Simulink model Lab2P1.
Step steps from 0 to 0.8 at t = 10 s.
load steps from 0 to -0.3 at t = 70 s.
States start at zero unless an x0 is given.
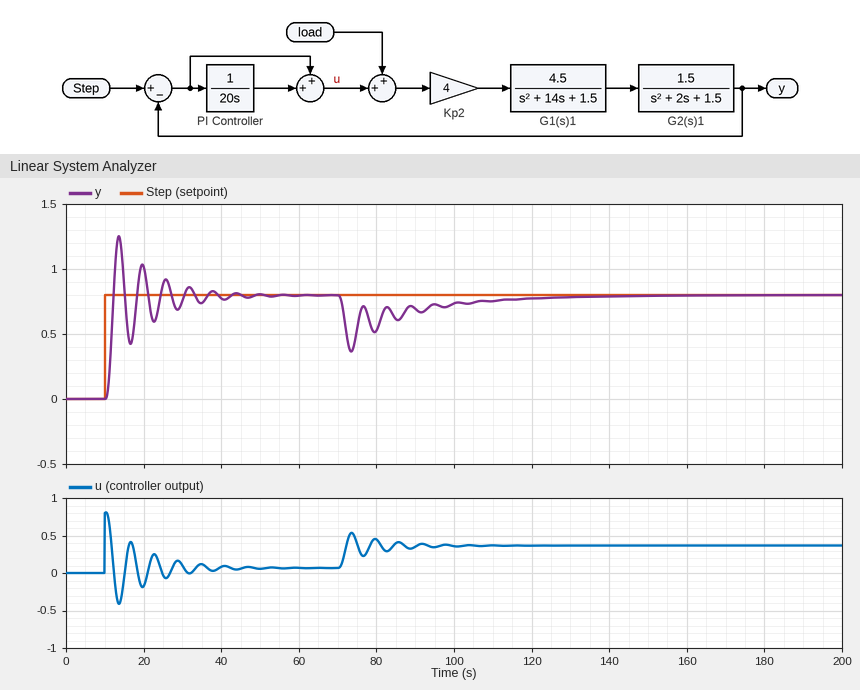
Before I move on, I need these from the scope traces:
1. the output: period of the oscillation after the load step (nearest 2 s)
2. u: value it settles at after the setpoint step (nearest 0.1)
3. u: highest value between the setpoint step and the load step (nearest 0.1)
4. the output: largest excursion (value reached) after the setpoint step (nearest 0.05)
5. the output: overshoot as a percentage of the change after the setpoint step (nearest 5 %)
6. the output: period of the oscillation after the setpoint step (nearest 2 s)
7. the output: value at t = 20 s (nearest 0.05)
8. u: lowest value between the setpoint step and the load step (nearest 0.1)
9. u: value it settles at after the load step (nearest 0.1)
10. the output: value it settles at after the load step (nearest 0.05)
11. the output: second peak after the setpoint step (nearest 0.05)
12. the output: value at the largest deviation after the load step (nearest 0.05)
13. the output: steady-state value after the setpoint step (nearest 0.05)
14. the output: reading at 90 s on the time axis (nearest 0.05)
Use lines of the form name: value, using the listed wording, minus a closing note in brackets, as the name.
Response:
the output: period of the oscillation after the load step: 6 s
u: value it settles at after the setpoint step: 0.1
u: highest value between the setpoint step and the load step: 0.8
the output: largest excursion (value reached) after the setpoint step: 1.25
the output: overshoot as a percentage of the change after the setpoint step: 55 %
the output: period of the oscillation after the setpoint step: 6 s
the output: value at t = 20 s: 1.00
u: lowest value between the setpoint step and the load step: -0.4
u: value it settles at after the load step: 0.4
the output: value it settles at after the load step: 0.80
the output: second peak after the setpoint step: 1.05
the output: value at the largest deviation after the load step: 0.35
the output: steady-state value after the setpoint step: 0.80
the output: reading at 90 s on the time axis: 0.70
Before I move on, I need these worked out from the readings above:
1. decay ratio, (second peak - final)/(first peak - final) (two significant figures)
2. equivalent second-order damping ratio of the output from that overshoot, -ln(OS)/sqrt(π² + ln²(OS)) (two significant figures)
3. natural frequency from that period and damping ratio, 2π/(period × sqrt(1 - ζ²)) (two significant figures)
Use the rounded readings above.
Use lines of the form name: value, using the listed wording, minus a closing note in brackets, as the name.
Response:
decay ratio, (second peak - final)/(first peak - final): 0.56
equivalent second-order damping ratio of the output from that overshoot, -ln(OS)/sqrt(π² + ln²(OS)): 0.19
natural frequency from that period and damping ratio, 2π/(period × sqrt(1 - ζ²)): 1.1 rad/s
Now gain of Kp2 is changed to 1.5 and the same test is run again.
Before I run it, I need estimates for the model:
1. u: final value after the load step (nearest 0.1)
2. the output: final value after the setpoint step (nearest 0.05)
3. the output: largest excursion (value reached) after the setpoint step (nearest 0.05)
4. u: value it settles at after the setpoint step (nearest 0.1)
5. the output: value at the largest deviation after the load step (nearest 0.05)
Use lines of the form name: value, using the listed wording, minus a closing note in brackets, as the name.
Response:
u: final value after the load step: 0.5
the output: final value after the setpoint step: 0.80
the output: largest excursion (value reached) after the setpoint step: 0.85
u: value it settles at after the setpoint step: 0.2
the output: value at the largest deviation after the load step: 0.50
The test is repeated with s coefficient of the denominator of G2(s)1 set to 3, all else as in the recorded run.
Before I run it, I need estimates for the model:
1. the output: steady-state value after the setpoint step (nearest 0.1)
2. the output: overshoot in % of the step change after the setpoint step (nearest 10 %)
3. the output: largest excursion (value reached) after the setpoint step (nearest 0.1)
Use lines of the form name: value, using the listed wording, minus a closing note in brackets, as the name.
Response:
the output: steady-state value after the setpoint step: 0.8
the output: overshoot in % of the step change after the setpoint step: 50 %
the output: largest excursion (value reached) after the setpoint step: 1.2
